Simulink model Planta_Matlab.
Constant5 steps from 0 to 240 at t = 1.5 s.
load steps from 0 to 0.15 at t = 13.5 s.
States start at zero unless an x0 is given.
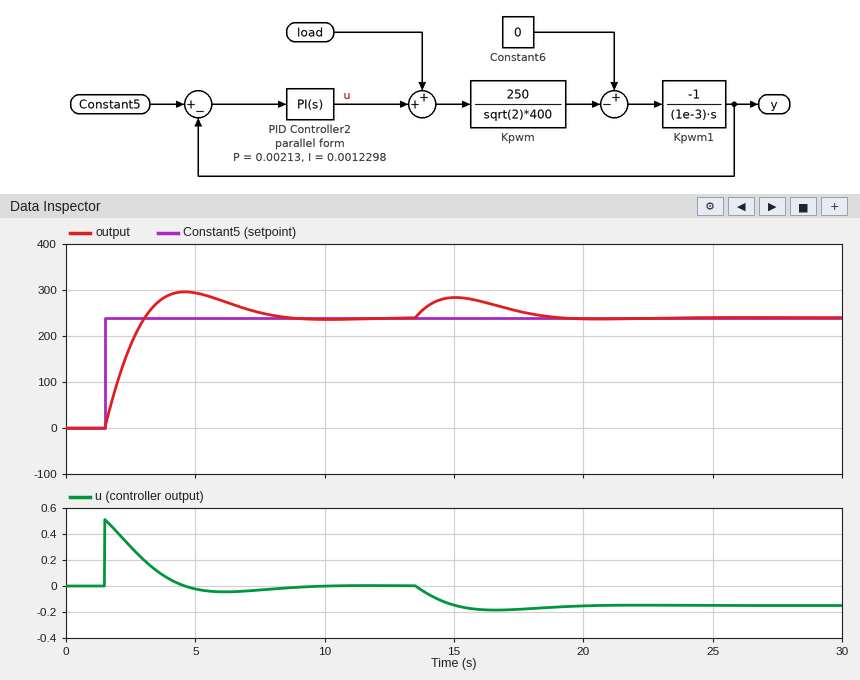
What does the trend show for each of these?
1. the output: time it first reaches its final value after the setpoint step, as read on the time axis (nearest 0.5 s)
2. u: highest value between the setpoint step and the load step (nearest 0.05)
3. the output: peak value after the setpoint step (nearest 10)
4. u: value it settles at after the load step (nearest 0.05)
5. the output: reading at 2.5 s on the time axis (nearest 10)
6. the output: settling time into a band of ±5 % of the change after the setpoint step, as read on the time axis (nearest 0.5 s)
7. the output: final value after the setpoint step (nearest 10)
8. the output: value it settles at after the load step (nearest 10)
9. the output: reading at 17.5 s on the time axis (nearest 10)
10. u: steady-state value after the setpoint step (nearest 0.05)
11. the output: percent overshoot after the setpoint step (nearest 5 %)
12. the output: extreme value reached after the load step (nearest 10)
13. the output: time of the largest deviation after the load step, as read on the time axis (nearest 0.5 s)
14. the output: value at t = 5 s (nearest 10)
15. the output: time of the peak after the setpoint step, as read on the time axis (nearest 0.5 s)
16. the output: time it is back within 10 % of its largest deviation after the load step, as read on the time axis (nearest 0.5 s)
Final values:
3.0 s
0.50
300
-0.15
180
7.5 s
240
240
250
0.00
25 %
280
15.0 s
290
4.5 s
18.5 s
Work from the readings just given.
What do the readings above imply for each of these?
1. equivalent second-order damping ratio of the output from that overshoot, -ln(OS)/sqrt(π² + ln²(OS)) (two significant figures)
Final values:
0.40
